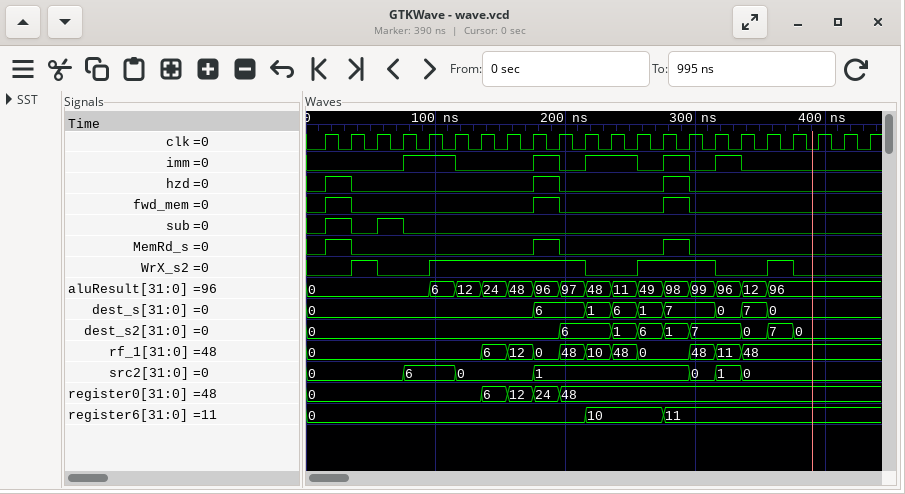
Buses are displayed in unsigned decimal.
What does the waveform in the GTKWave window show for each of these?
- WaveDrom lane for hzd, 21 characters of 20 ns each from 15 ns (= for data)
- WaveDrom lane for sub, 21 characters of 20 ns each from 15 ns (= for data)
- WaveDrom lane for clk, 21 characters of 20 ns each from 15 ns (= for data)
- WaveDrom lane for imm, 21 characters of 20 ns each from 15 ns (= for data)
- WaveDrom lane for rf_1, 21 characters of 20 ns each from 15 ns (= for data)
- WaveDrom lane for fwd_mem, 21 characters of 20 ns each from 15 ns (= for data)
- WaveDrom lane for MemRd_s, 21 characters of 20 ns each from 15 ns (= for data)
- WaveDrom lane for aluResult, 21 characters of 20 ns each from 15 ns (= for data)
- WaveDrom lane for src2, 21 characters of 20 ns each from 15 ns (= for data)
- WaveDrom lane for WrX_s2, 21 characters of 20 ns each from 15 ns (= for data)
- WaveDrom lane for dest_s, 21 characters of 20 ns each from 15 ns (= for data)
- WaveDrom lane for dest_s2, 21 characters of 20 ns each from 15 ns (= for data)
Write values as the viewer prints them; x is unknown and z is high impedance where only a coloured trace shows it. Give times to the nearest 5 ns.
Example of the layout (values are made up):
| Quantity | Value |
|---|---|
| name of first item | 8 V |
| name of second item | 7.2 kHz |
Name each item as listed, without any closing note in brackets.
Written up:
| Quantity | Value |
|---|---|
| WaveDrom lane for hzd, 21 characters of 20 ns each from 15 ns | {name: 'hzd', wave: '10......10...10......'} |
| WaveDrom lane for sub, 21 characters of 20 ns each from 15 ns | {name: 'sub', wave: '1010.................'} |
| WaveDrom lane for clk, 21 characters of 20 ns each from 15 ns | {name: 'clk', wave: 'p....................'} |
| WaveDrom lane for imm, 21 characters of 20 ns each from 15 ns | {name: 'imm', wave: '0..1.0..101.01010....'} |
| WaveDrom lane for rf_1, 21 characters of 20 ns each from 15 ns | {name: 'rf_1', wave: '=.....=======.===....', data: '0 6 12 0 48 10 48 0 48 11 48'} |
| WaveDrom lane for fwd_mem, 21 characters of 20 ns each from 15 ns | {name: 'fwd_mem', wave: '10......10...10......'} |
| WaveDrom lane for MemRd_s, 21 characters of 20 ns each from 15 ns | {name: 'MemRd_s', wave: '10......10...10......'} |
| WaveDrom lane for aluResult, 21 characters of 20 ns each from 15 ns | {name: 'aluResult', wave: '=...==============...', data: '0 6 12 24 48 96 97 48 11 49 98 99 96 12 96'} |
| WaveDrom lane for src2, 21 characters of 20 ns each from 15 ns | {name: 'src2', wave: '=..=.=..=.....===....', data: '0 6 0 1 0 1 0'} |
| WaveDrom lane for WrX_s2, 21 characters of 20 ns each from 15 ns | {name: 'WrX_s2', wave: '010.1.....0.1..0.10..'} |
| WaveDrom lane for dest_s, 21 characters of 20 ns each from 15 ns | {name: 'dest_s', wave: '=.......=.====.===...', data: '0 6 1 6 1 7 0 7 0'} |
| WaveDrom lane for dest_s2, 21 characters of 20 ns each from 15 ns | {name: 'dest_s2', wave: '=........=.====.===..', data: '0 6 1 6 1 7 0 7 0'} |
